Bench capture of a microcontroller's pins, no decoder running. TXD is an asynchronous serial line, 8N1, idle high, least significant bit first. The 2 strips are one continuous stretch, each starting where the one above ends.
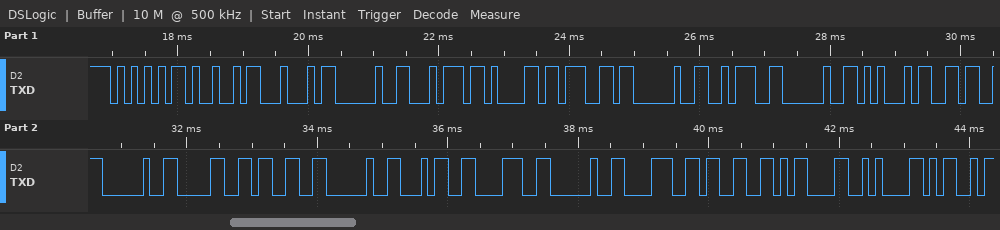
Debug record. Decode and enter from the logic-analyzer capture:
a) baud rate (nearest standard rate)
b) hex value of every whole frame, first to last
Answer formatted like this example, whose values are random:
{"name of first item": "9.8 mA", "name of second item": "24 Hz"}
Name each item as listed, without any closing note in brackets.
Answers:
{"baud rate": "9600 baud", "hex value of every whole frame, first to last": "55 49 44 20 74 61 67 20 3A 20 45 36 20 30 33 20 34 38 20 38 33 0D 0A 4D"}
